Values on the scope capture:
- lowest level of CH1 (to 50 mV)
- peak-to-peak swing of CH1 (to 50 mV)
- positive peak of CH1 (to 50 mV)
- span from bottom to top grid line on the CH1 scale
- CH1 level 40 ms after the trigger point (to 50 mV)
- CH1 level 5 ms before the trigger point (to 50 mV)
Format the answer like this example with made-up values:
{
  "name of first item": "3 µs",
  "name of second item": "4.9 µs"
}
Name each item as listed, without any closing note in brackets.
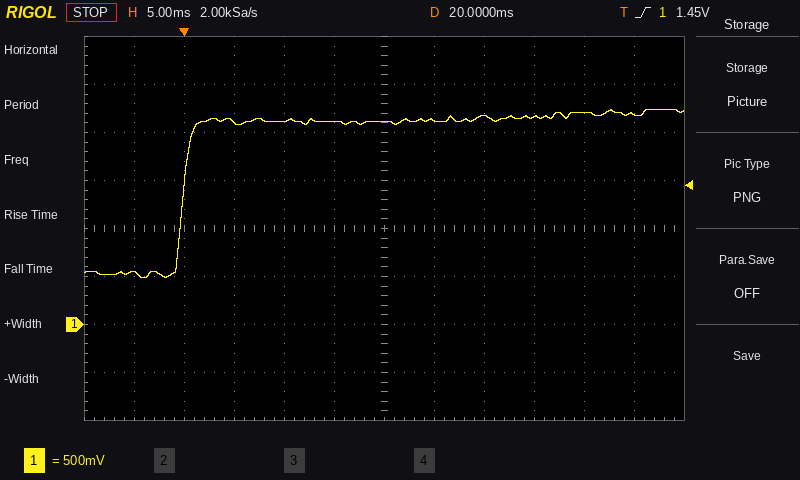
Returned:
{
  "lowest level of CH1": "500 mV",
  "peak-to-peak swing of CH1": "1.75 V",
  "positive peak of CH1": "2.25 V",
  "span from bottom to top grid line on the CH1 scale": "4 V",
  "CH1 level 40 ms after the trigger point": "2.20 V",
  "CH1 level 5 ms before the trigger point": "550 mV"
}
